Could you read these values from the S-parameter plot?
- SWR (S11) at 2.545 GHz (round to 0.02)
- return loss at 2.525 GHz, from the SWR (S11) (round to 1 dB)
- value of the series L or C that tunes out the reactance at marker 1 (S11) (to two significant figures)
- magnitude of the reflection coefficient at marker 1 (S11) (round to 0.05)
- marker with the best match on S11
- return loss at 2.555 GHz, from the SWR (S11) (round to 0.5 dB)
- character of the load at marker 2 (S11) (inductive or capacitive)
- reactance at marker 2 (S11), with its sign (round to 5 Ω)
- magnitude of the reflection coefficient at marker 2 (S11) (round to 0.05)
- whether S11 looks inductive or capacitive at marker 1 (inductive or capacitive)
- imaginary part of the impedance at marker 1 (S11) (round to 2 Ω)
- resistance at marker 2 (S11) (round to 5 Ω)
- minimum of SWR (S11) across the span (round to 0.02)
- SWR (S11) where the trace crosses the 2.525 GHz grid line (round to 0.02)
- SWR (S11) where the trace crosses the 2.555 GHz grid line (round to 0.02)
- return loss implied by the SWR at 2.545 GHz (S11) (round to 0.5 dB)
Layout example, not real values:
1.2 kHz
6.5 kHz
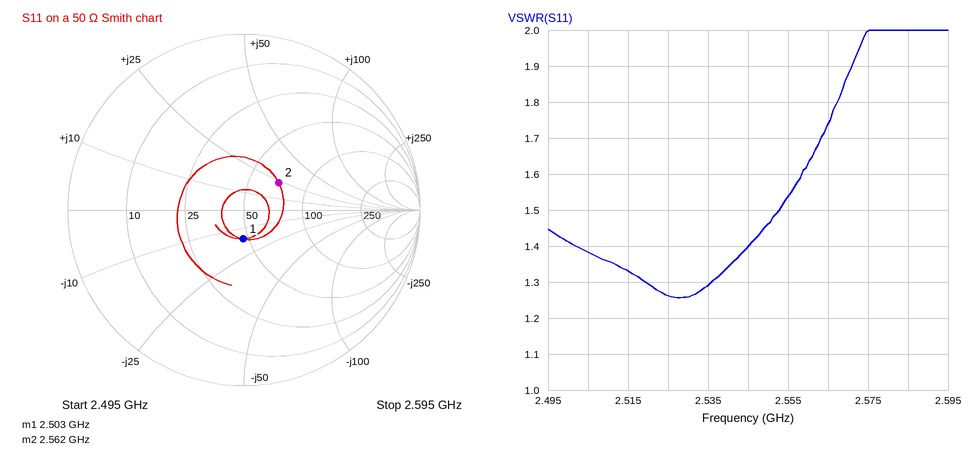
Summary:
1.40
19 dB
1.0 nH
0.15
marker 1
13.5 dB
inductive
+25 Ω
0.25
capacitive
-16 Ω
70 Ω
1.26
1.26
1.54
15.5 dB
